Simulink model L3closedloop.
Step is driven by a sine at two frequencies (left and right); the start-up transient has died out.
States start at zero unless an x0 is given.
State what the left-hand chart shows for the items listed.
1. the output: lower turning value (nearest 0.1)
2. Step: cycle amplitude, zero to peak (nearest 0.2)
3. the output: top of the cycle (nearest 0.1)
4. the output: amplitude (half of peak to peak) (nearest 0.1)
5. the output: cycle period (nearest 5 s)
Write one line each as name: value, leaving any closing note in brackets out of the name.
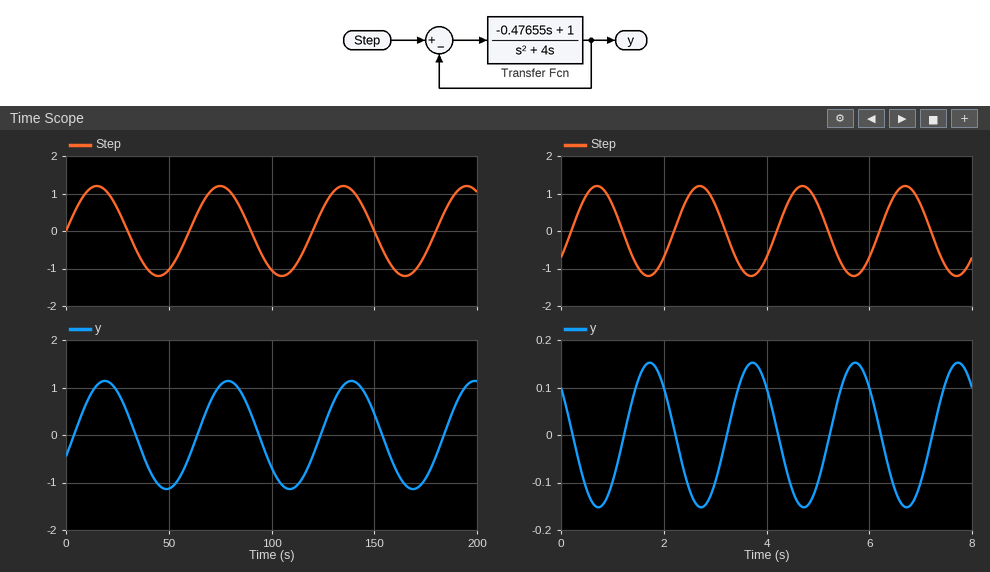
the output: lower turning value: -1.1
Step: cycle amplitude, zero to peak: 1.2
the output: top of the cycle: 1.1
the output: amplitude (half of peak to peak): 1.1
the output: cycle period: 60 s
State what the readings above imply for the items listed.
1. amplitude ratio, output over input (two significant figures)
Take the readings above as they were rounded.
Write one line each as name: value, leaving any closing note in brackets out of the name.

amplitude ratio, output over input: 0.92
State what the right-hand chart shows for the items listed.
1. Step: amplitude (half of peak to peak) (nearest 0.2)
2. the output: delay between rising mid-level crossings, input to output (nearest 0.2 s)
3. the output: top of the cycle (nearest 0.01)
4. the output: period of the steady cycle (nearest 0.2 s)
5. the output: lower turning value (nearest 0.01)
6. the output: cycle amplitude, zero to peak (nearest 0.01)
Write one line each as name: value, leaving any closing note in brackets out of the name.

Step: amplitude (half of peak to peak): 1.2
the output: delay between rising mid-level crossings, input to output: 1.0 s
the output: top of the cycle: 0.15
the output: period of the steady cycle: 2.0 s
the output: lower turning value: -0.15
the output: cycle amplitude, zero to peak: 0.15
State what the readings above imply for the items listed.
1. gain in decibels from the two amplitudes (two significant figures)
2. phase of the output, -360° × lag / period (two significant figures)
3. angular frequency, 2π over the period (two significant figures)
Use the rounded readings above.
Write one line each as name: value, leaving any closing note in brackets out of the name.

gain in decibels from the two amplitudes: -18 dB
phase of the output, -360° × lag / period: -180°
angular frequency, 2π over the period: 3.1 rad/s
